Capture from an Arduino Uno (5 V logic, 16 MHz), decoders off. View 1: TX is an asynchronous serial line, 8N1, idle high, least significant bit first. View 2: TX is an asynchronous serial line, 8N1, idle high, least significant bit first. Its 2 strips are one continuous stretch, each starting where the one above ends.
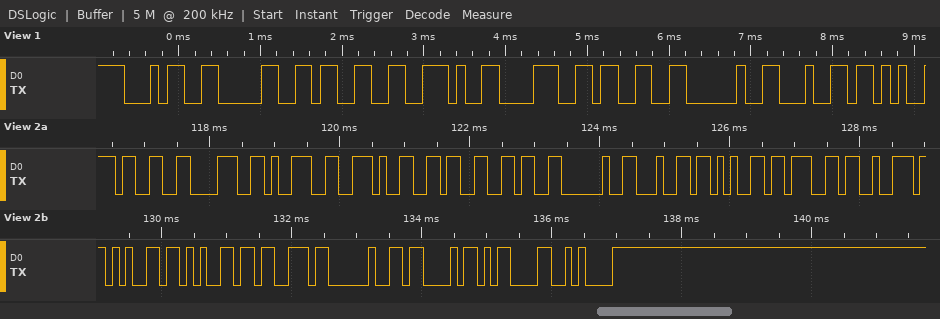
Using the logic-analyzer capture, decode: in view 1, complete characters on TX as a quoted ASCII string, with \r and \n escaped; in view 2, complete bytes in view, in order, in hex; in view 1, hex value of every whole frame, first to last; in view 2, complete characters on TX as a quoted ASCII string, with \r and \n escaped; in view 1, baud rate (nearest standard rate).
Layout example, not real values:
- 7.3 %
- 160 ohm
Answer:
- "403.83 d"
- 0x33 0x38 0x39 0x2E 0x36 0x36 0x20 0x64 0x65 0x67 0x72 0x65 0x65 0x73 0x20 0x43 0x0D 0x0A
- 34 30 33 2E 38 33 20 64
- "389.66 degrees C\r\n"
- 9600 baud
